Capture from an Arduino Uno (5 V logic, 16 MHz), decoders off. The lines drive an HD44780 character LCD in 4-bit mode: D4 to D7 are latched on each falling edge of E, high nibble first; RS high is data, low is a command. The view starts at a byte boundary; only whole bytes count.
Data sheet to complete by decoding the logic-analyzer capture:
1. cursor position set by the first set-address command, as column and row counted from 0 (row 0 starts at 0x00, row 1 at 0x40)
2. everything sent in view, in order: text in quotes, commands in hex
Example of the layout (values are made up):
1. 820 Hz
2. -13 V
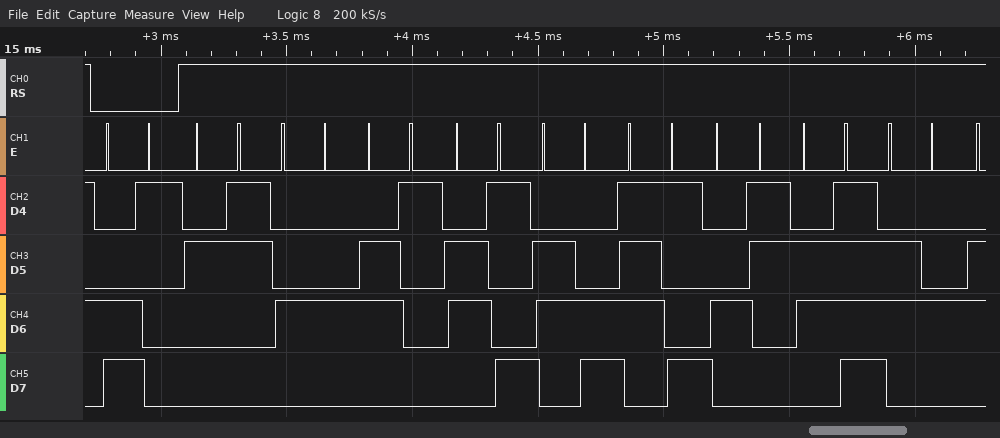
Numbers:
1. column 1, row 1
2. 0xC1 "#DailyCod"
